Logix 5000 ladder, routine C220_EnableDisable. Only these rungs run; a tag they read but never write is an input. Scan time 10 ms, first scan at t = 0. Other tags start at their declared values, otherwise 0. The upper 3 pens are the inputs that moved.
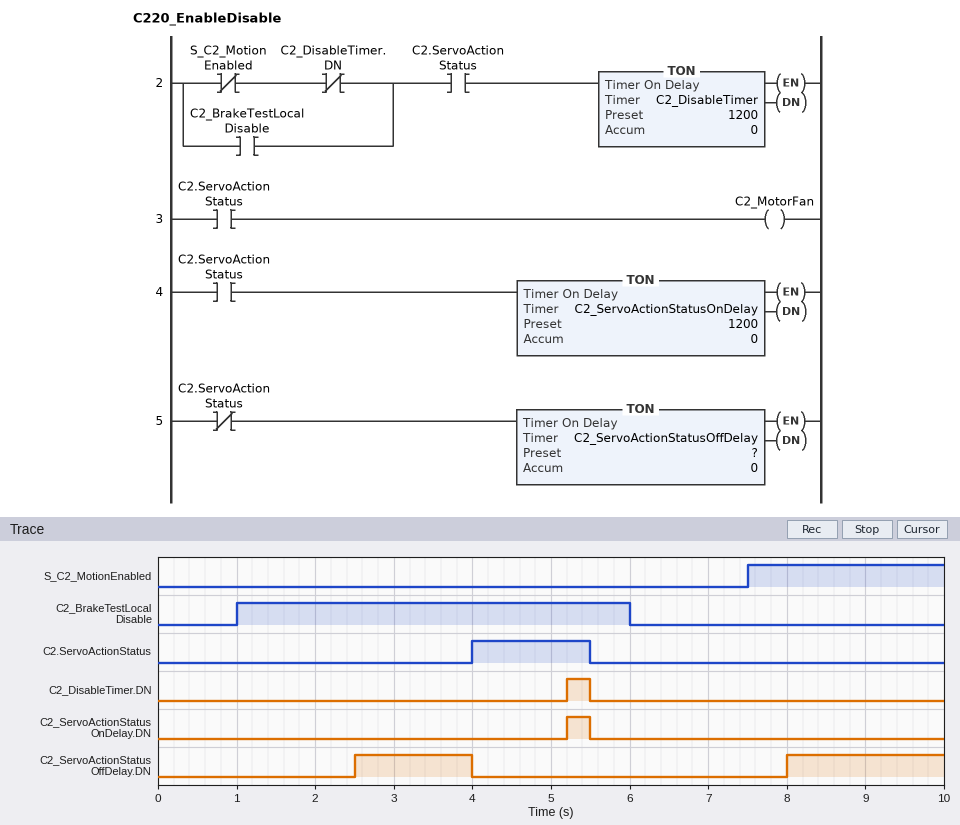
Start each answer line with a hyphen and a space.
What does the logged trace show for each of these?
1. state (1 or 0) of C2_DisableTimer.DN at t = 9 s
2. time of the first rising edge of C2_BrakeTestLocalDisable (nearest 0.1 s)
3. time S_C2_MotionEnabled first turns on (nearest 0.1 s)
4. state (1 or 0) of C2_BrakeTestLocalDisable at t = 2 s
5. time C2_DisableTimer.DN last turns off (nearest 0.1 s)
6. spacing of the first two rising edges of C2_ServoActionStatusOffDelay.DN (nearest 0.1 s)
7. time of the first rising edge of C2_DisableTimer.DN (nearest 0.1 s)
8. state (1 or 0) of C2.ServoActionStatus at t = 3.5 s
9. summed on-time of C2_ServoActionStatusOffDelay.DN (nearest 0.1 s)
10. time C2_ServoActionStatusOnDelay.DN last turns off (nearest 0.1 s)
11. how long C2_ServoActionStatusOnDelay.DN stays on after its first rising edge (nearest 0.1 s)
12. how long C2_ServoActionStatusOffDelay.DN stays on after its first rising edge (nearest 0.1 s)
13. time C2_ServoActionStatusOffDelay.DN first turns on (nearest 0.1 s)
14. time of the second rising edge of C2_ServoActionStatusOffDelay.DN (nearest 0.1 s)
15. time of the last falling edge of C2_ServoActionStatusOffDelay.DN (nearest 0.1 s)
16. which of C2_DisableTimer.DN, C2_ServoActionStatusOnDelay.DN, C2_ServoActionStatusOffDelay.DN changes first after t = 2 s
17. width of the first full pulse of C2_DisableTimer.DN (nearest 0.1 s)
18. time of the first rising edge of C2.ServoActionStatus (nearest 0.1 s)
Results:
- 0
- 1.0 s
- 7.5 s
- 1
- 5.5 s
- 5.5 s
- 5.2 s
- 0
- 3.5 s
- 5.5 s
- 0.3 s
- 1.5 s
- 2.5 s
- 8.0 s
- 4.0 s
- C2_ServoActionStatusOffDelay.DN
- 0.3 s
- 4.0 s
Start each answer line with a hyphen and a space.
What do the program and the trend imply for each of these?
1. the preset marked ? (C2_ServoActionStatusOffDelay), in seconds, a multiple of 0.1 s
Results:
- 2.5 s
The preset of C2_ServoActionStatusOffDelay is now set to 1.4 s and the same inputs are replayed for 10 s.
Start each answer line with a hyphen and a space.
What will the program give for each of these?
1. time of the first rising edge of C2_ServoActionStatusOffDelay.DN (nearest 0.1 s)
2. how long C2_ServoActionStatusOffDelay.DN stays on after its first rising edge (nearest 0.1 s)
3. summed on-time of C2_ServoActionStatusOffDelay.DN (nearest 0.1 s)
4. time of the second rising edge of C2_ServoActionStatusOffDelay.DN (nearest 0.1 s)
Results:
- 1.4 s
- 2.6 s
- 5.7 s
- 6.9 s
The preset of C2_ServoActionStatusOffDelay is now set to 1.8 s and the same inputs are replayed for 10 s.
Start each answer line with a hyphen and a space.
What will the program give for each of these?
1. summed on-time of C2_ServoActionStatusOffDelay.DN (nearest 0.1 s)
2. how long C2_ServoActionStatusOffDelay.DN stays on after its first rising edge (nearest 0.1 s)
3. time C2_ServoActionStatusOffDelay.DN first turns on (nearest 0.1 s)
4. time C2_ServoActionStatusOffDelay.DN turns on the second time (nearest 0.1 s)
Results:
- 4.9 s
- 2.2 s
- 1.8 s
- 7.3 s
